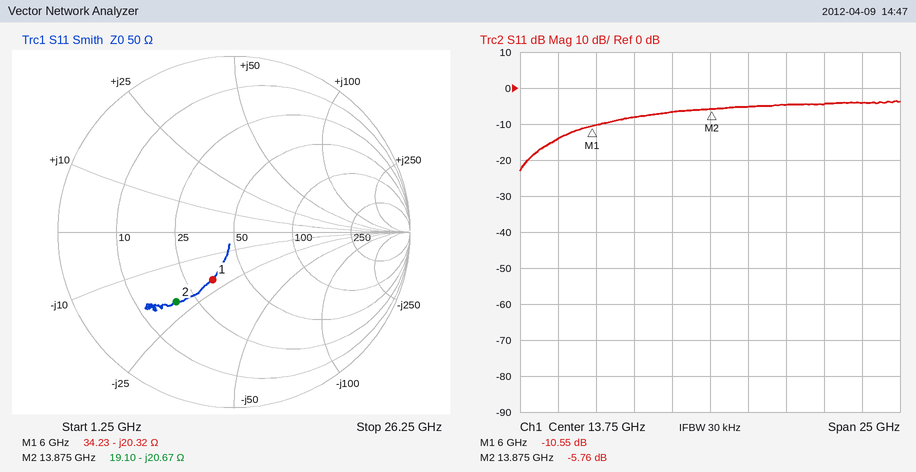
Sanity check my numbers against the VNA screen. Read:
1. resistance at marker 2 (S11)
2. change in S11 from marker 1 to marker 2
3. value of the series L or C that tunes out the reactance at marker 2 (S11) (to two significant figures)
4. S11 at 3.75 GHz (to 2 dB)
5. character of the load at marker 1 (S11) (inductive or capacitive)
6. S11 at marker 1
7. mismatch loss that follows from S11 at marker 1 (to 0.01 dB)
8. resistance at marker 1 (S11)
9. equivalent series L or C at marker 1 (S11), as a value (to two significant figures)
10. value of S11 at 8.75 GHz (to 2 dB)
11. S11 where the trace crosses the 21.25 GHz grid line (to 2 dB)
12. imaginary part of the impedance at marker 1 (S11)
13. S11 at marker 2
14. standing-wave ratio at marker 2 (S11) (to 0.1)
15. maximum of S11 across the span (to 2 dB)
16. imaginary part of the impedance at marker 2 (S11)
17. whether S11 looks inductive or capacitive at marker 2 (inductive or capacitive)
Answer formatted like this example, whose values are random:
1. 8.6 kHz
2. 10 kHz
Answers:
1. 19.10 Ω
2. 4.79 dB
3. 240 pH
4. -14 dB
5. capacitive
6. -10.55 dB
7. 0.40 dB
8. 34.23 Ω
9. 1.3 pF
10. -8 dB
11. -4 dB
12. -20.32 Ω
13. -5.76 dB
14. 3.1
15. -4 dB
16. -20.67 Ω
17. capacitive
